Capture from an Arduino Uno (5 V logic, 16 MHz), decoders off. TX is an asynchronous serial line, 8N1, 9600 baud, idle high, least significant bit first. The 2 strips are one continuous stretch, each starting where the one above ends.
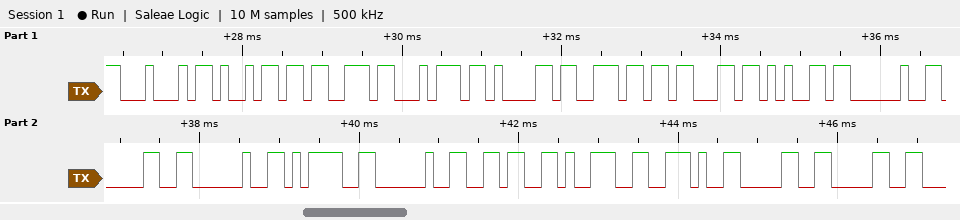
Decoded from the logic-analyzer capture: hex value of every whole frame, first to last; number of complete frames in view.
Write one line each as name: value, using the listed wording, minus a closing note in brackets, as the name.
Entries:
hex value of every whole frame, first to last: 0x44 0x69 0x73 0x74 0x61 0x6E 0x63 0x65 0x20 0x30 0x20 0x3D 0x20 0x36 0x39 0x2E 0x30 0x30
number of complete frames in view: 18
